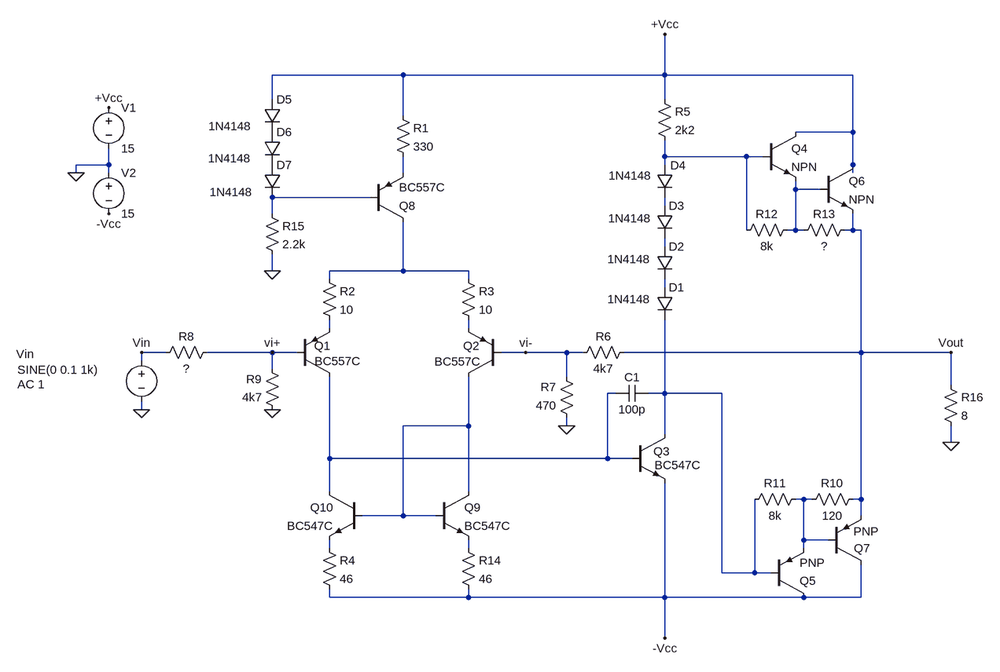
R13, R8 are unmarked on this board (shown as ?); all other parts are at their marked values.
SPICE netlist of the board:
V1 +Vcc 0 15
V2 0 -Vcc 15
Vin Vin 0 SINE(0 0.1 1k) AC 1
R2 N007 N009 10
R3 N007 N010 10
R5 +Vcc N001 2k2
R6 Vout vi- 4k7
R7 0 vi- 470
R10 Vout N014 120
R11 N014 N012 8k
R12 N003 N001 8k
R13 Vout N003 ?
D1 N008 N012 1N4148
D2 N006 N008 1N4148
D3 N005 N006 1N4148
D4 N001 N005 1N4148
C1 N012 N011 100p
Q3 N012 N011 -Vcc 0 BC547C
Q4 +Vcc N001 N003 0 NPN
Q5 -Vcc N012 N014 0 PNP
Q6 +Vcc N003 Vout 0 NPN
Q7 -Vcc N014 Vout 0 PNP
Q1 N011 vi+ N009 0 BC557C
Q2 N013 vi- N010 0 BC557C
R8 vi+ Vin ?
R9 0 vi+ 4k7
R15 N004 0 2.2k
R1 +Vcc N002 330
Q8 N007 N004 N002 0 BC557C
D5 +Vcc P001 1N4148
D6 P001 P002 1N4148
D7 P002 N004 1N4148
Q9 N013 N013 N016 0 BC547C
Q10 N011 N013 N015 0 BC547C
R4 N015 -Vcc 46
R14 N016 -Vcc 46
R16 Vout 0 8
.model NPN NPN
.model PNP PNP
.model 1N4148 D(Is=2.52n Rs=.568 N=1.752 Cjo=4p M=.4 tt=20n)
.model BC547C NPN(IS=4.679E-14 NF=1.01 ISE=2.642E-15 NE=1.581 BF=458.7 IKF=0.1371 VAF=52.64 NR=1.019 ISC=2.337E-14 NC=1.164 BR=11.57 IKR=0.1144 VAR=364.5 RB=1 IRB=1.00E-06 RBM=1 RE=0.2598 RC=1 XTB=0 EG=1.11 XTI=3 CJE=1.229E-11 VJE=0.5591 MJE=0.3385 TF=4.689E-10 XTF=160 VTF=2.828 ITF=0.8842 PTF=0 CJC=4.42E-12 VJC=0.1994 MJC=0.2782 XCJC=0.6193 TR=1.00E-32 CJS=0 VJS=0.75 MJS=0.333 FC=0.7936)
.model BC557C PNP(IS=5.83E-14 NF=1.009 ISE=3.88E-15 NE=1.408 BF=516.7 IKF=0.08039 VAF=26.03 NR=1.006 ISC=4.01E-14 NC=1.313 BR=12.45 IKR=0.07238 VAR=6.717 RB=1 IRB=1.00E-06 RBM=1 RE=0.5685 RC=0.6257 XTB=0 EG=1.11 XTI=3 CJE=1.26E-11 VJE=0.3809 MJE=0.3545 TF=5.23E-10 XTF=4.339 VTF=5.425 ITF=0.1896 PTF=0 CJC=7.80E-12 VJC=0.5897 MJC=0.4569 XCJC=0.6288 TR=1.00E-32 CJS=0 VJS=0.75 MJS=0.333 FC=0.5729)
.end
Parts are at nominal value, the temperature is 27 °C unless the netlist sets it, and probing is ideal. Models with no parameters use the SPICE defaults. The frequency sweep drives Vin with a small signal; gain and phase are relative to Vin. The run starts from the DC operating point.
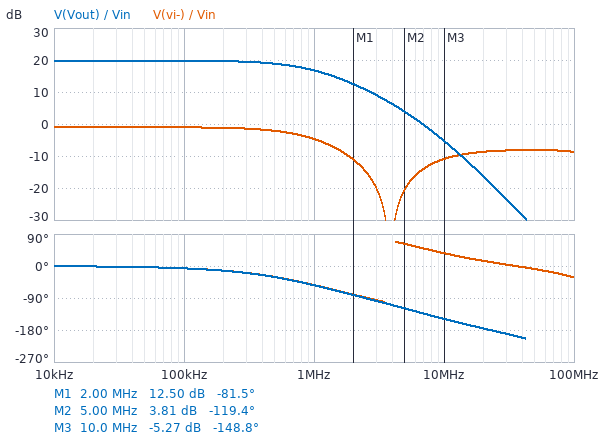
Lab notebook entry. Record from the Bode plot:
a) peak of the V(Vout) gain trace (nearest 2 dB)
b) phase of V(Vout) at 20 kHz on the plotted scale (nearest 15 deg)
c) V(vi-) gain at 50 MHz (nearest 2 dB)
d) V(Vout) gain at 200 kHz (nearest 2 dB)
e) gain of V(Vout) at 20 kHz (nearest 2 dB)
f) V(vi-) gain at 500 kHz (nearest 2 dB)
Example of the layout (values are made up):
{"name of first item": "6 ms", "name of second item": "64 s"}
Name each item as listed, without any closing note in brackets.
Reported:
{"peak of the V(Vout) gain trace": "20 dB", "phase of V(Vout) at 20 kHz on the plotted scale": "0 deg", "V(vi-) gain at 50 MHz": "-8 dB", "V(Vout) gain at 200 kHz": "20 dB", "gain of V(Vout) at 20 kHz": "20 dB", "V(vi-) gain at 500 kHz": "-2 dB"}
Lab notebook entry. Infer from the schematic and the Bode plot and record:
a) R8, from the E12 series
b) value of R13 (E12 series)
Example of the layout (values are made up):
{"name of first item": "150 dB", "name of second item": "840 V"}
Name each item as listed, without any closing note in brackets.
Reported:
{"R8, from the E12 series": "560 Ω", "value of R13": "68 Ω"}
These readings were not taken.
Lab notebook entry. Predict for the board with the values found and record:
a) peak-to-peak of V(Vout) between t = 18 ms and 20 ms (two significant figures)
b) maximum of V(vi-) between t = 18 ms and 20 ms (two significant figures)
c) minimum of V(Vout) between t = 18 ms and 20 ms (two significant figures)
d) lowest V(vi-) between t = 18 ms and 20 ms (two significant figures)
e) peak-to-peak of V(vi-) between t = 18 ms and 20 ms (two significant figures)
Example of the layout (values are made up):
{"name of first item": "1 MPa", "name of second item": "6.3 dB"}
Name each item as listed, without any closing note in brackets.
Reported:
{"peak-to-peak of V(Vout) between t = 18 ms and 20 ms": "2.0 V", "maximum of V(vi-) between t = 18 ms and 20 ms": "91 mV", "minimum of V(Vout) between t = 18 ms and 20 ms": "-980 mV", "lowest V(vi-) between t = 18 ms and 20 ms": "-88 mV", "peak-to-peak of V(vi-) between t = 18 ms and 20 ms": "180 mV"}
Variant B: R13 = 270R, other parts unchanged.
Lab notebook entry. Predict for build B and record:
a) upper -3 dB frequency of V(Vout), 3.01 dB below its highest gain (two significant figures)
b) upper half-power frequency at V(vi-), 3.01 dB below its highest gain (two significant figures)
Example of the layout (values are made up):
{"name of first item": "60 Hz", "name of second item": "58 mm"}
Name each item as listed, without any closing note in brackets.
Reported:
{"upper -3 dB frequency of V(Vout), 3.01 dB below its highest gain": "990 kHz", "upper half-power frequency at V(vi-), 3.01 dB below its highest gain": "890 kHz"}
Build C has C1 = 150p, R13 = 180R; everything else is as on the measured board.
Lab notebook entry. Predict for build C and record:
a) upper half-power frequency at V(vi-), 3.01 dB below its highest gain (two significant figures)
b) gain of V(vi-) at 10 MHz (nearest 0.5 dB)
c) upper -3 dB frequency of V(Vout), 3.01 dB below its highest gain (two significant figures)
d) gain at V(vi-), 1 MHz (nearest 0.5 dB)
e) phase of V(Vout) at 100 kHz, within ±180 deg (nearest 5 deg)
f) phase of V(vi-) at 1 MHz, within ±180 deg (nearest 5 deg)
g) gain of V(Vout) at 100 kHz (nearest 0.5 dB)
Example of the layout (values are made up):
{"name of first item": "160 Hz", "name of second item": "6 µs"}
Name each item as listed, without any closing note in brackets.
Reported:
{"upper half-power frequency at V(vi-), 3.01 dB below its highest gain": "380 kHz", "gain of V(vi-) at 10 MHz": "-10.5 dB", "upper -3 dB frequency of V(Vout), 3.01 dB below its highest gain": "400 kHz", "gain at V(vi-), 1 MHz": "-11.0 dB", "phase of V(Vout) at 100 kHz, within ±180 deg": "-15 deg", "phase of V(vi-) at 1 MHz, within ±180 deg": "-75 deg", "gain of V(Vout) at 100 kHz": "19.5 dB"}
